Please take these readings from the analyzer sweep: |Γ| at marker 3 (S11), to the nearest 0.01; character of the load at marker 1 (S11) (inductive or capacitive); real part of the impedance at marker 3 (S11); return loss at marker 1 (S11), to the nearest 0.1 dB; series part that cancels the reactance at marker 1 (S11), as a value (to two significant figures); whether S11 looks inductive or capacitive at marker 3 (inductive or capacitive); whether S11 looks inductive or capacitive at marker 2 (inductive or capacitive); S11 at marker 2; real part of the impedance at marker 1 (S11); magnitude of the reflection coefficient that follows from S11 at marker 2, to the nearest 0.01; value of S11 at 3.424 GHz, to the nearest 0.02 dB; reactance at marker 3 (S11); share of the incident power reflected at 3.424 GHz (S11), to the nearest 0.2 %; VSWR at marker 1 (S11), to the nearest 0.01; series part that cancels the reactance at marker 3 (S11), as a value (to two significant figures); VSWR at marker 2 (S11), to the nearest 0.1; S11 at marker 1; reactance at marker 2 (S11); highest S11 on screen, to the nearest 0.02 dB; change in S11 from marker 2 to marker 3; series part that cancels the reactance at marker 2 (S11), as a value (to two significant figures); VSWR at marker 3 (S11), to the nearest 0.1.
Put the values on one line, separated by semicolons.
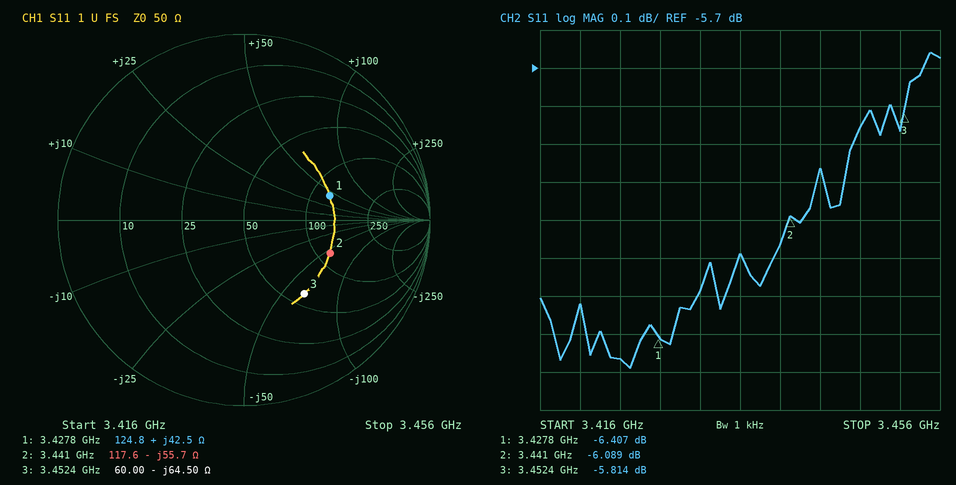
0.51; inductive; 60.00 Ω; 6.4 dB; 1.1 pF; capacitive; capacitive; -6.089 dB; 124.8 Ω; 0.50; -6.46 dB; -64.50 Ω; 22.6 %; 2.83; 3.0 nH; 3.0; -6.407 dB; -55.7 Ω; -5.66 dB; 0.275 dB; 2.6 nH; 3.1
